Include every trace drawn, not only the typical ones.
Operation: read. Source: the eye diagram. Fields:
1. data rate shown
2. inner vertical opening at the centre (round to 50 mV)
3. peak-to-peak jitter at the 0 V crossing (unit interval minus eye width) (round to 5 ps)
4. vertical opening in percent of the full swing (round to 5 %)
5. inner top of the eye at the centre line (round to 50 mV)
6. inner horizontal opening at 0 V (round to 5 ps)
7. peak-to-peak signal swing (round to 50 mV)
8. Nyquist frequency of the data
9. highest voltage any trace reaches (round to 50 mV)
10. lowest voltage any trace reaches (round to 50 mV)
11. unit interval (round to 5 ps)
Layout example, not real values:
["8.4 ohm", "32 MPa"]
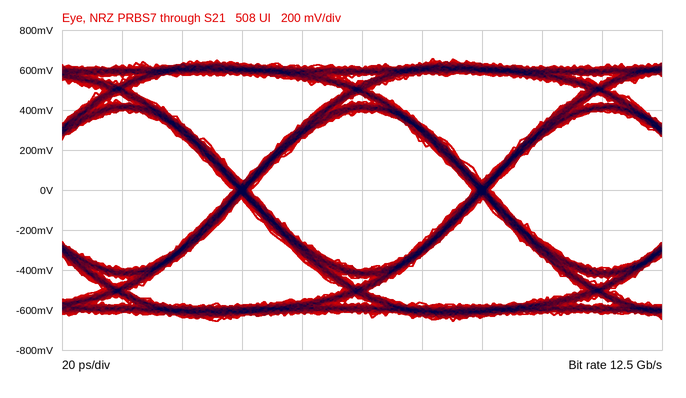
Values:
["12.5 Gb/s", "800 mV", "5 ps", "60 %", "400 mV", "75 ps", "1.30 V", "6.25 GHz", "650 mV", "-650 mV", "80 ps"]
